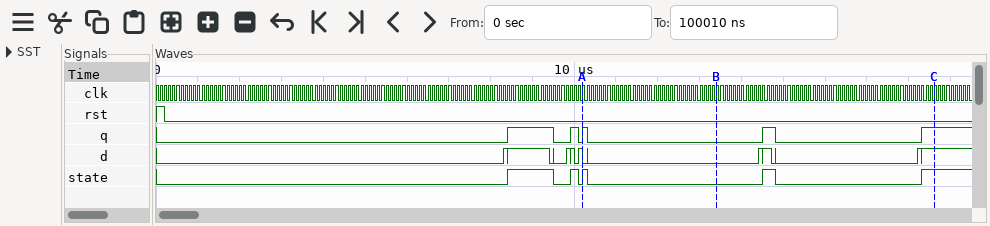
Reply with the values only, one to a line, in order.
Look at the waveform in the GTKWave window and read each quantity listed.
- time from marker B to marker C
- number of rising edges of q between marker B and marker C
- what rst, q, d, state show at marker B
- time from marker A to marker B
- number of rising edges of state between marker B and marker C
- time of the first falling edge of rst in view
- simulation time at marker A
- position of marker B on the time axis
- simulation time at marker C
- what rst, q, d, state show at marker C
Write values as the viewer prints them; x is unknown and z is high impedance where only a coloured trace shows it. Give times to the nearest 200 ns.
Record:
5200 ns
2
rst=0, q=0, d=0, state=0
3200 ns
2
200 ns
10200 ns
13400 ns
18600 ns
rst=0, q=1, d=1, state=1
